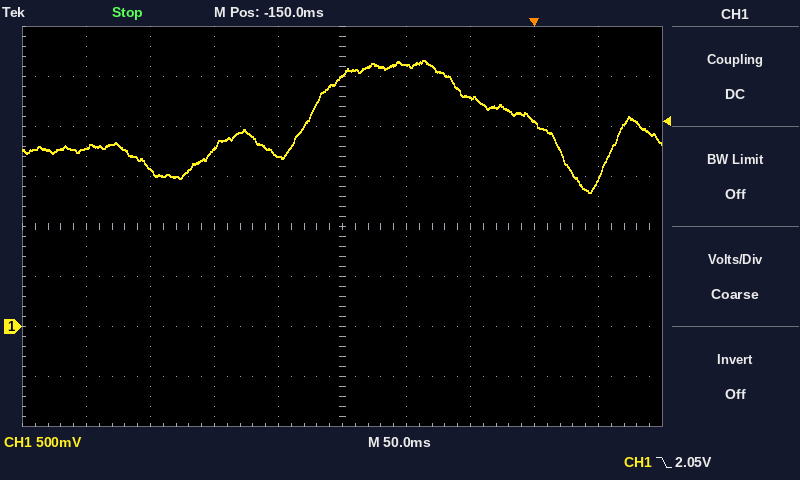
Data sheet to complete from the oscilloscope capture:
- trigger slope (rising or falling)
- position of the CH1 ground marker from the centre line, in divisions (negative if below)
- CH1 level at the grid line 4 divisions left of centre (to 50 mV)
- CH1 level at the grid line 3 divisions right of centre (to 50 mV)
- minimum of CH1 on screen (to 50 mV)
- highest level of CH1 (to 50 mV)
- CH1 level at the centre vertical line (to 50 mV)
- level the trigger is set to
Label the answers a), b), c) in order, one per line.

a) falling
b) -2.0 div
c) 1.80 V
d) 2.05 V
e) 1.35 V
f) 2.65 V
g) 2.50 V
h) 2.05 V
